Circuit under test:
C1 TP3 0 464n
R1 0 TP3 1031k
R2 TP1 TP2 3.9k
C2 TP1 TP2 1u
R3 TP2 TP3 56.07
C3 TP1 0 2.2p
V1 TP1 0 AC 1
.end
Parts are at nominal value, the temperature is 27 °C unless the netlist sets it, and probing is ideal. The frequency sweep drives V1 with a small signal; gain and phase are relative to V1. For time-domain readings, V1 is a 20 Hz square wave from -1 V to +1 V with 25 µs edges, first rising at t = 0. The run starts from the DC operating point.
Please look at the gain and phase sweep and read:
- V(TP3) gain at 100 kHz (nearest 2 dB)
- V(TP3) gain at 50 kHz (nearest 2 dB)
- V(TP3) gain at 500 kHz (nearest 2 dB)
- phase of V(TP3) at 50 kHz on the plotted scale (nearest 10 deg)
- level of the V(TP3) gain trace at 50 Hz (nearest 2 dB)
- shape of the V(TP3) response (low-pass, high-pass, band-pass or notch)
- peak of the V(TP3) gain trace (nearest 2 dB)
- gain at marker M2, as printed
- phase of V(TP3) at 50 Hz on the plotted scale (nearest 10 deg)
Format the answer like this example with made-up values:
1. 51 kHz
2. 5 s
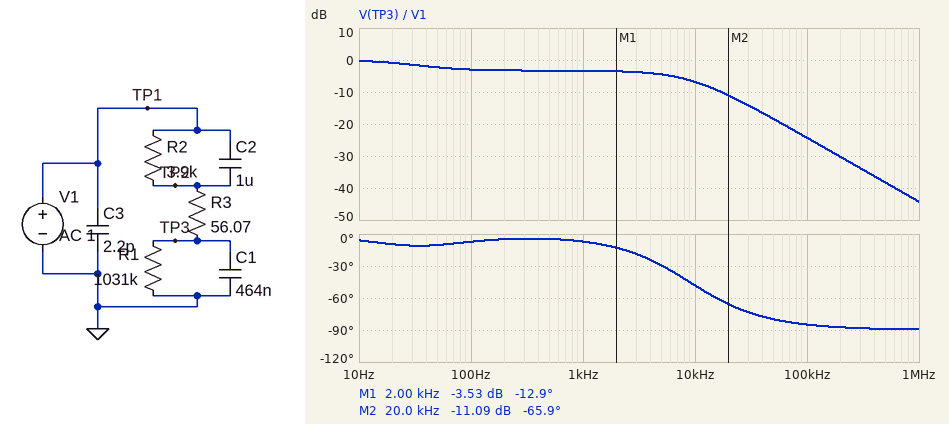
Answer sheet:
1. -24 dB
2. -18 dB
3. -38 dB
4. -80 deg
5. -2 dB
6. low-pass
7. 0 dB
8. -11.09 dB
9. -10 deg
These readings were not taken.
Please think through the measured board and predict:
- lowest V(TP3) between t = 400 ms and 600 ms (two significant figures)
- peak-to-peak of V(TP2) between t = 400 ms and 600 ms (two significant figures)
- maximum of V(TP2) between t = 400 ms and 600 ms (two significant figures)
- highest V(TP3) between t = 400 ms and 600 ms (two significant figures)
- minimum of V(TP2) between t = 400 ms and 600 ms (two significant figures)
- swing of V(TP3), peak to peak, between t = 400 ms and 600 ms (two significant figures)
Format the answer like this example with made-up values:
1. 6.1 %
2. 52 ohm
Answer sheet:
1. -990 mV
2. 2.0 V
3. 990 mV
4. 990 mV
5. -990 mV
6. 2.0 V
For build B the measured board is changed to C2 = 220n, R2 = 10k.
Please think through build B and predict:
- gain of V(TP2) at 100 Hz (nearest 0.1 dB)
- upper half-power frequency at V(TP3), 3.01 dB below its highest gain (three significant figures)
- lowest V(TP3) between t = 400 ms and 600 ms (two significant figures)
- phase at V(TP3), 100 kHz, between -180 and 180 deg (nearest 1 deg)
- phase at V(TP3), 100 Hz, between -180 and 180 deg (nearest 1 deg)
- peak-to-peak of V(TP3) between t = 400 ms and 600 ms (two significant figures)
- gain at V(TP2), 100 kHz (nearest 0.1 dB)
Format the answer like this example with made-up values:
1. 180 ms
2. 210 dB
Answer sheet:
1. -8.3 dB
2. 26.4 Hz
3. -960 mV
4. -79 deg
5. -23 deg
6. 1.9 V
7. -0.1 dB
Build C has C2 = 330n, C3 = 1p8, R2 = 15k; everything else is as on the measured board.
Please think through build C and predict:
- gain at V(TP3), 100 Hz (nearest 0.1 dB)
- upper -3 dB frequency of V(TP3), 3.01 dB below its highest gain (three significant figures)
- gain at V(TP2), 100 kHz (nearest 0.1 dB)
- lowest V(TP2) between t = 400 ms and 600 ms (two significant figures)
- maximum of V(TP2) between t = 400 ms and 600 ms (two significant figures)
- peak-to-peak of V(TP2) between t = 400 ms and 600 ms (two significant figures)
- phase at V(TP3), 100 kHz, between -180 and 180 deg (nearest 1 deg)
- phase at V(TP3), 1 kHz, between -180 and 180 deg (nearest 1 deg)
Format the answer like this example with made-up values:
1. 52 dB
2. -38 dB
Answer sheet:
1. -7.3 dB
2. 16.9 Hz
3. -0.1 dB
4. -860 mV
5. 860 mV
6. 1.7 V
7. -82 deg
8. -5 deg
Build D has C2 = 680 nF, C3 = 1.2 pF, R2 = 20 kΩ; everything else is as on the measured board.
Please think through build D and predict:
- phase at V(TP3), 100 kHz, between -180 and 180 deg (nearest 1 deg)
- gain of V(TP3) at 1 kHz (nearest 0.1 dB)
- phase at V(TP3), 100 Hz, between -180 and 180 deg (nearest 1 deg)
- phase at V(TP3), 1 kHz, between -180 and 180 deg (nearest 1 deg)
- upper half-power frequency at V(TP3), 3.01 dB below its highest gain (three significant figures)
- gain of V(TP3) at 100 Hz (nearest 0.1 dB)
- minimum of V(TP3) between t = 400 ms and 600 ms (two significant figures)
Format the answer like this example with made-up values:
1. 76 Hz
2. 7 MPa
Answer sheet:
1. -84 deg
2. -4.6 dB
3. -3 deg
4. -6 deg
5. 13.7 Hz
6. -4.5 dB
7. -790 mV
